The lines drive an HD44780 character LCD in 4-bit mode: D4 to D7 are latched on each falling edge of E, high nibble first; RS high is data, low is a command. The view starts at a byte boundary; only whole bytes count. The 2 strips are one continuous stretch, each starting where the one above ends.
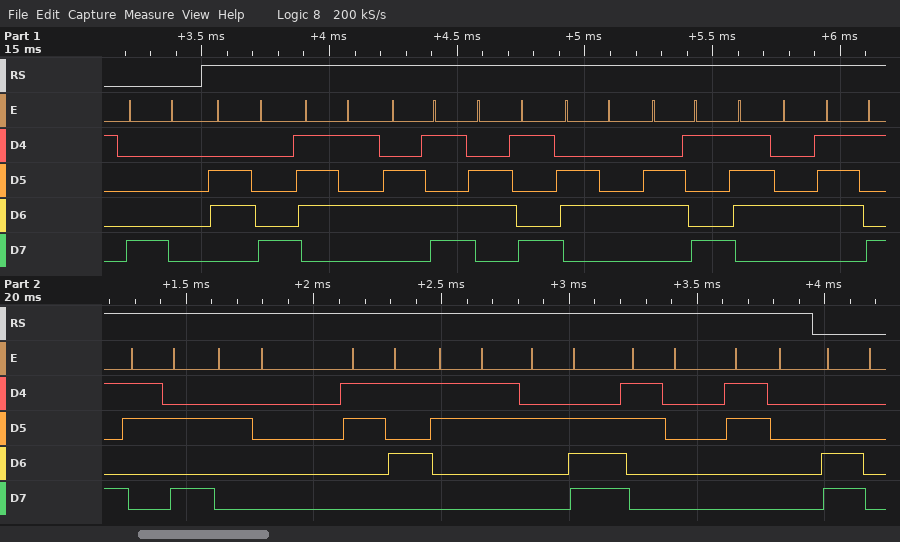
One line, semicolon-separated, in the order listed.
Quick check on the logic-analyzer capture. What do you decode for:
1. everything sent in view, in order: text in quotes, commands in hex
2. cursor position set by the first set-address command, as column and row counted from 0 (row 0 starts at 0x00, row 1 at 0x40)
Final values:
0x80 "humidity: 53.00" 0xC0; column 0, row 0
